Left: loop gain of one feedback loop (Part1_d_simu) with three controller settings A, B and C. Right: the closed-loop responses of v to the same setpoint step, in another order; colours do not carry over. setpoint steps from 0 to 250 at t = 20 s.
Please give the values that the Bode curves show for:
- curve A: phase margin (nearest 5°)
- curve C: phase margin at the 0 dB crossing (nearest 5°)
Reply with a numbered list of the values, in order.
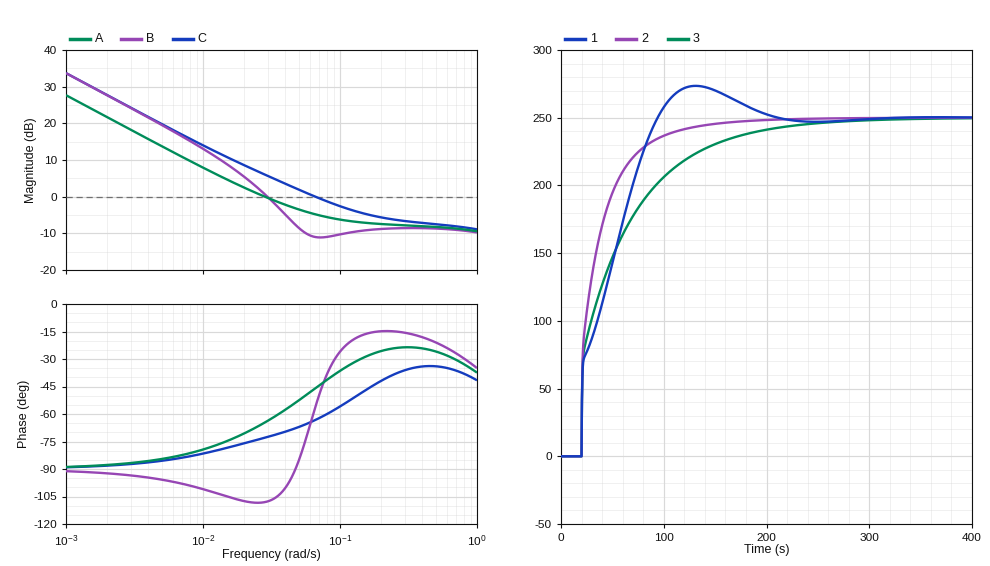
1. 115°
2. 115°
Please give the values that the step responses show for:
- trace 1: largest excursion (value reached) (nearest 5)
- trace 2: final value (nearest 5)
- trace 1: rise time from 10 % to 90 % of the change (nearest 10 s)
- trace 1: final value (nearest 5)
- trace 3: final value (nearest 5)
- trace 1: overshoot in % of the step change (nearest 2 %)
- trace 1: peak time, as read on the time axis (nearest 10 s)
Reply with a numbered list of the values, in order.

1. 275
2. 250
3. 60 s
4. 250
5. 250
6. 10 %
7. 130 s
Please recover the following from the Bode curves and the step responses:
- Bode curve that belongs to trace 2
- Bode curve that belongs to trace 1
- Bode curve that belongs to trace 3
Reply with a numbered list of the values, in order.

1. C
2. B
3. A
